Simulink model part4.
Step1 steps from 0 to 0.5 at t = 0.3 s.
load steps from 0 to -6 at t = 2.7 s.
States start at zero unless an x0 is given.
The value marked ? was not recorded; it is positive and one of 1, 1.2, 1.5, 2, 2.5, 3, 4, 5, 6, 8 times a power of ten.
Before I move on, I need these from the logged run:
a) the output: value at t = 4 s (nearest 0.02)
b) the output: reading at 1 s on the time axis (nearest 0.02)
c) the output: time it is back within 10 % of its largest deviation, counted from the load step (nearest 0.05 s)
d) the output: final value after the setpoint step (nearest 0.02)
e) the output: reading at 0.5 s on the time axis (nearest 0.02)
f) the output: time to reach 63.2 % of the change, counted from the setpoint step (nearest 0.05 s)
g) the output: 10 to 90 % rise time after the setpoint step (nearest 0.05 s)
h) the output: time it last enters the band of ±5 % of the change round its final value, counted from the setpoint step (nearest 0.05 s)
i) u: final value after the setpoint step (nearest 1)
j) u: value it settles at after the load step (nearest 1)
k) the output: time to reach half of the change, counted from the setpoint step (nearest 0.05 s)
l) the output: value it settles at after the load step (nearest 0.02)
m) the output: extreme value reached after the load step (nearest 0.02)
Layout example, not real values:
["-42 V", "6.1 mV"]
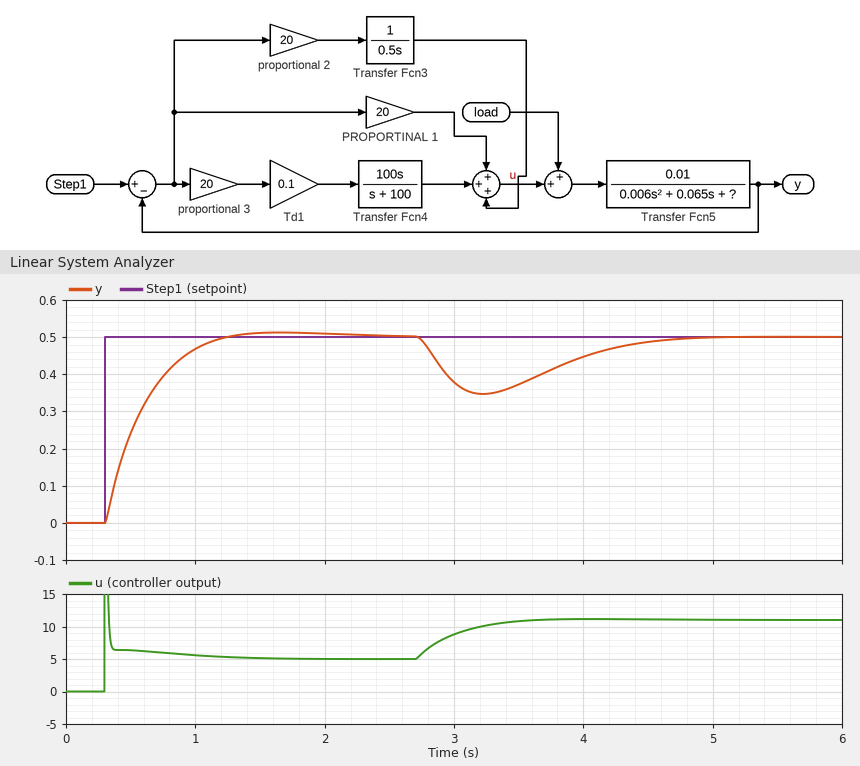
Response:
["0.44", "0.46", "1.75 s", "0.50", "0.24", "0.30 s", "0.60 s", "0.75 s", "5", "11", "0.20 s", "0.50", "0.34"]
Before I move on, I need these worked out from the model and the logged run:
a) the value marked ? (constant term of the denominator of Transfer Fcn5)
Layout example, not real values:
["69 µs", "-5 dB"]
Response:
["0.1"]
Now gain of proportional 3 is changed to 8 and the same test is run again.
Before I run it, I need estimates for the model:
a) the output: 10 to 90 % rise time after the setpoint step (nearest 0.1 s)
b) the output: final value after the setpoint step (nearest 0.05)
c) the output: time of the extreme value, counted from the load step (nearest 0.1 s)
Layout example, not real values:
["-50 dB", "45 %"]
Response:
["0.5 s", "0.50", "0.5 s"]
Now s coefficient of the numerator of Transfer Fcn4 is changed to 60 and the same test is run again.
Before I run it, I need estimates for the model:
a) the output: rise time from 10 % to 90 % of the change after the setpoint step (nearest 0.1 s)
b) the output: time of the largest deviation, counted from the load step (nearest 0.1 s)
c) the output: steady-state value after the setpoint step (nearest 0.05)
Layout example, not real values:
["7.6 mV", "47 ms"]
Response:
["0.5 s", "0.5 s", "0.50"]
